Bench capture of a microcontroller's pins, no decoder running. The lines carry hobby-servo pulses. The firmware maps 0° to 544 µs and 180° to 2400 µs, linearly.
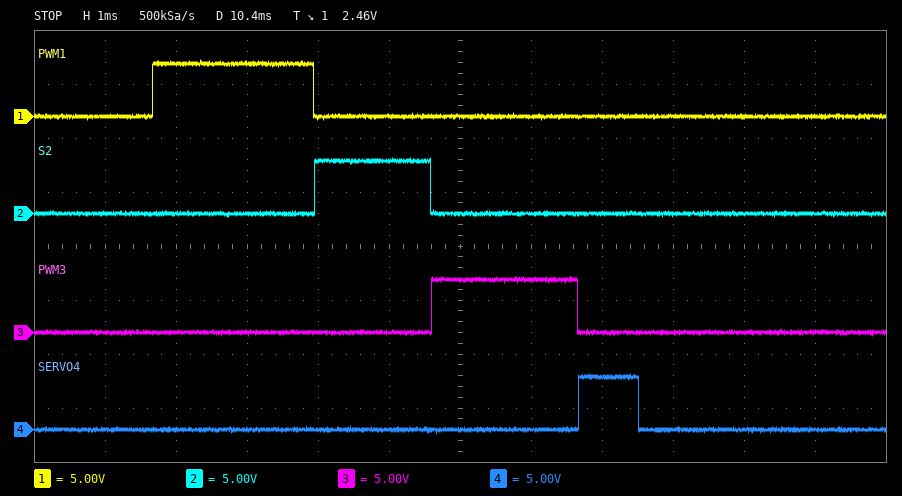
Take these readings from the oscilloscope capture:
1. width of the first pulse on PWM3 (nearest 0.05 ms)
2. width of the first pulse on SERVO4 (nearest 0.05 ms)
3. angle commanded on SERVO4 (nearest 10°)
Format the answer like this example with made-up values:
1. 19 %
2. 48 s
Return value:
1. 2.05 ms
2. 0.85 ms
3. 30°
